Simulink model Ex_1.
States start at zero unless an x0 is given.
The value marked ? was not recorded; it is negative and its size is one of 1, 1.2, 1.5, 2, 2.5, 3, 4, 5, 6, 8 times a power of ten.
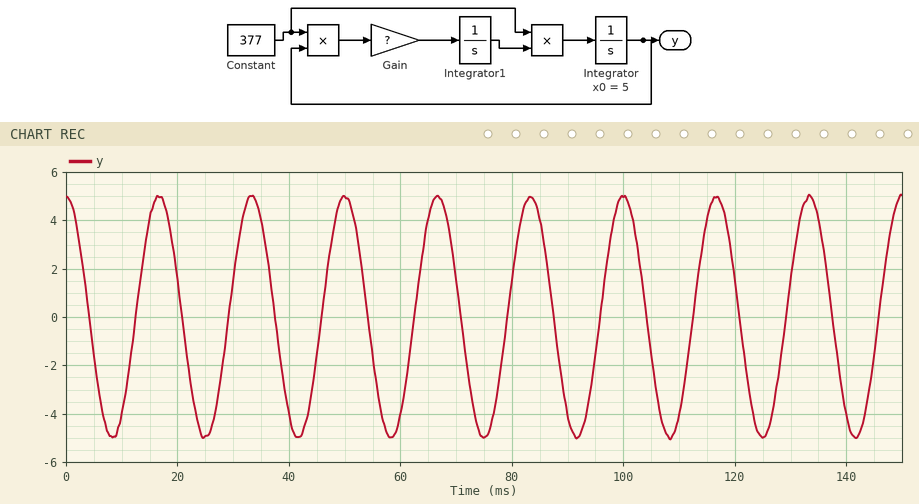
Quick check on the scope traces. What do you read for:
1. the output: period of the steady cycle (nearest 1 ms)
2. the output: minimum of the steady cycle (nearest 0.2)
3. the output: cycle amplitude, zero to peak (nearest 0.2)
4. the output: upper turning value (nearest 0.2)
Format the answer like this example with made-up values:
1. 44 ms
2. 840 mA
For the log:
1. 17 ms
2. -5.0
3. 5.0
4. 5.0
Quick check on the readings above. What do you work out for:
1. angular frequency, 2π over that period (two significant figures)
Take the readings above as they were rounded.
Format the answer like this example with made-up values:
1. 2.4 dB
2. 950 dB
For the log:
1. 0.37 rad/ms
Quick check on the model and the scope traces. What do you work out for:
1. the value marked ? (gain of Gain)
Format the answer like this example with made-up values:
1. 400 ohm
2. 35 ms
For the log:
1. -1
